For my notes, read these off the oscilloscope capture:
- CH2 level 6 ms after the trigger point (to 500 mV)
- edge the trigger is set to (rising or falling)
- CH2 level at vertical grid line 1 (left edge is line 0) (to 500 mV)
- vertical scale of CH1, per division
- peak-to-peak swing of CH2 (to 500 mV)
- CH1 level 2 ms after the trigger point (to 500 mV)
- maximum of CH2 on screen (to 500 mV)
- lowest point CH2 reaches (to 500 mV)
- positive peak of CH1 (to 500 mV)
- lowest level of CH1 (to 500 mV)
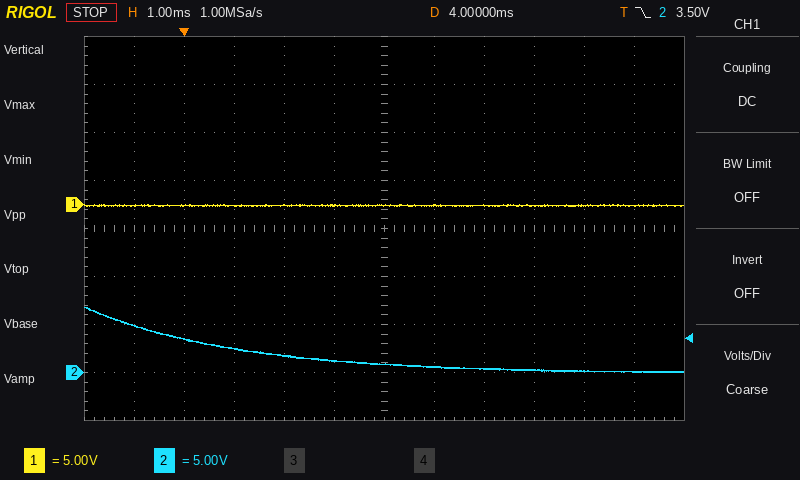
500 mV
falling
5.0 V
5 V
7.0 V
0.0 V
7.0 V
0.0 V
0.0 V
0.0 V
